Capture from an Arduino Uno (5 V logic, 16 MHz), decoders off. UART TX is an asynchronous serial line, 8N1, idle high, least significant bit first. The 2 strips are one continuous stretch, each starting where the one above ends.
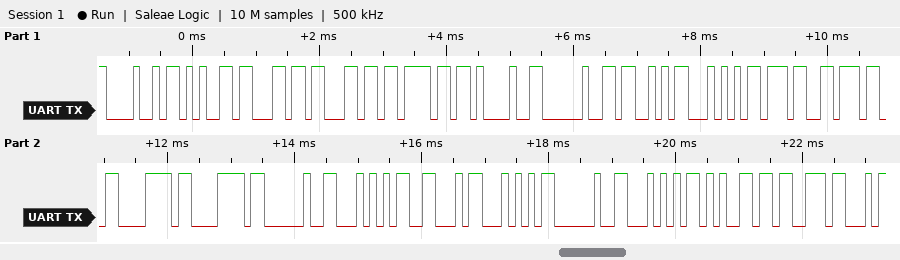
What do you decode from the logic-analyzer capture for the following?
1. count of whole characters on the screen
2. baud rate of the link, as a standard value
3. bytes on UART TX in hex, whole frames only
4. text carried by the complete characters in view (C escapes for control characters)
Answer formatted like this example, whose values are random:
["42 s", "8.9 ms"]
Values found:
["21", "9600 baud", "0x48 0x65 0x6C 0x6C 0x6F 0x21 0x20 0x53 0x54 0x37 0x37 0x78 0x78 0x20 0x54 0x46 0x54 0x20 0x54 0x65 0x73", "\"Hello! ST77xx TFT Tes\""]
